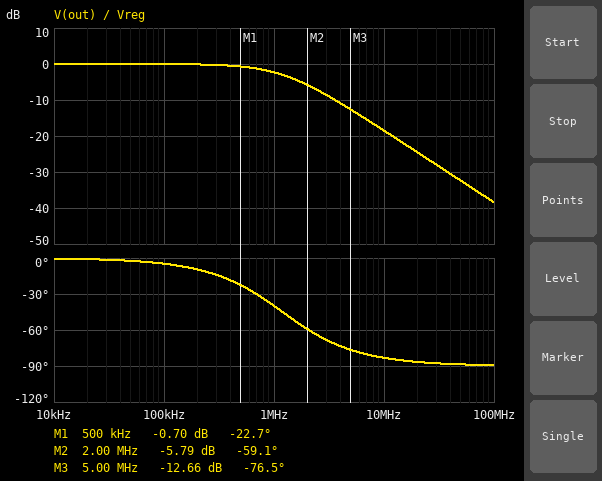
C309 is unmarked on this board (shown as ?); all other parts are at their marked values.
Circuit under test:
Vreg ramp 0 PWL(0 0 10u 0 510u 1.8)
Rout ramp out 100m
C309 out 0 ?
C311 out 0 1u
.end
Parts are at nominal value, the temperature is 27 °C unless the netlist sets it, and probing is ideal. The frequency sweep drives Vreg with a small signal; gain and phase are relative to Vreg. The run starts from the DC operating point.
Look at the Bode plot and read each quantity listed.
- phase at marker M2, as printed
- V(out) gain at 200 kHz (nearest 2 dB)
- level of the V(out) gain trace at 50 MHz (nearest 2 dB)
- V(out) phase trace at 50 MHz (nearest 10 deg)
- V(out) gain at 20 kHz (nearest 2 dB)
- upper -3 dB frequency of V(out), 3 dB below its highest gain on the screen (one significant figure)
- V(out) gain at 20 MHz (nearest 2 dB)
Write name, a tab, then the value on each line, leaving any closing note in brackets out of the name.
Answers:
phase at marker M2, as printed	-59.1 deg
V(out) gain at 200 kHz	0 dB
level of the V(out) gain trace at 50 MHz	-32 dB
V(out) phase trace at 50 MHz	-90 deg
V(out) gain at 20 kHz	0 dB
upper -3 dB frequency of V(out), 3 dB below its highest gain on the screen	1 MHz
V(out) gain at 20 MHz	-24 dB
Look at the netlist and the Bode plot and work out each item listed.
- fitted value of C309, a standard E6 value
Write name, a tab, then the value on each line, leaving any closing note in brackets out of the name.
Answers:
fitted value of C309, a standard E6 value	330 nF
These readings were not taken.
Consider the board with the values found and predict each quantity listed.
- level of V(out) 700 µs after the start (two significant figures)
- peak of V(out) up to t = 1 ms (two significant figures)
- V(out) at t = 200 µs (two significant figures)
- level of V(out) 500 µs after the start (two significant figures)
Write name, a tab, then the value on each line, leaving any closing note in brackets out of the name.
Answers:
level of V(out) 700 µs after the start	1.8 V
peak of V(out) up to t = 1 ms	1.8 V
V(out) at t = 200 µs	680 mV
level of V(out) 500 µs after the start	1.8 V
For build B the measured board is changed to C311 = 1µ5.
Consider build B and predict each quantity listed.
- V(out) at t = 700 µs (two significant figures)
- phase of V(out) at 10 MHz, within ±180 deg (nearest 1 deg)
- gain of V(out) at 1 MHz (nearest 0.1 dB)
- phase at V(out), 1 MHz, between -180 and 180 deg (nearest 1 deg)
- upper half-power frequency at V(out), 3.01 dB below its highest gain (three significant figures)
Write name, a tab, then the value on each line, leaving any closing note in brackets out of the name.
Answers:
V(out) at t = 700 µs	1.8 V
phase of V(out) at 10 MHz, within ±180 deg	-85 deg
gain of V(out) at 1 MHz	-3.7 dB
phase at V(out), 1 MHz, between -180 and 180 deg	-49 deg
upper half-power frequency at V(out), 3.01 dB below its highest gain	870 kHz
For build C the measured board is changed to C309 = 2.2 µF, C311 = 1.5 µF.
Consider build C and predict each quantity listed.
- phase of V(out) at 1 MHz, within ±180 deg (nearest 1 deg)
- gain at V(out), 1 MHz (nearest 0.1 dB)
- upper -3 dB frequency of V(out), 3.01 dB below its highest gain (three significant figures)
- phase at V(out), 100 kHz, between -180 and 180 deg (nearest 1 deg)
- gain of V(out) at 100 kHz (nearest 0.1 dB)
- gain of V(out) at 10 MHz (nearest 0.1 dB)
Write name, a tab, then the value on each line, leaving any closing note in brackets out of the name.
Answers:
phase of V(out) at 1 MHz, within ±180 deg	-67 deg
gain at V(out), 1 MHz	-8.1 dB
upper -3 dB frequency of V(out), 3.01 dB below its highest gain	430 kHz
phase at V(out), 100 kHz, between -180 and 180 deg	-13 deg
gain of V(out) at 100 kHz	-0.2 dB
gain of V(out) at 10 MHz	-27.3 dB
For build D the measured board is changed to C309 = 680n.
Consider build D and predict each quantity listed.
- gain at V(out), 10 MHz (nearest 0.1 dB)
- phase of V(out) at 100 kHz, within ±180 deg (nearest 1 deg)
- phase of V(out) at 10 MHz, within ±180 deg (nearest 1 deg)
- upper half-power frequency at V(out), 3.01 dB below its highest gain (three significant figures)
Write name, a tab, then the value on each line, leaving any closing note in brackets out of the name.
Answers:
gain at V(out), 10 MHz	-20.5 dB
phase of V(out) at 100 kHz, within ±180 deg	-6 deg
phase of V(out) at 10 MHz, within ±180 deg	-85 deg
upper half-power frequency at V(out), 3.01 dB below its highest gain	947 kHz
